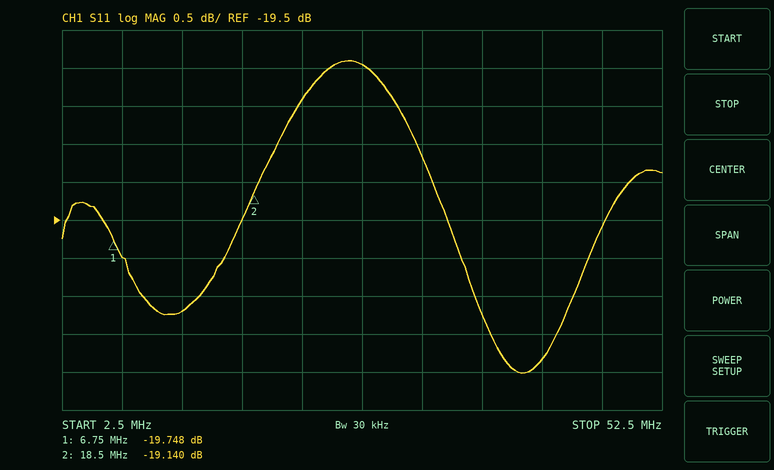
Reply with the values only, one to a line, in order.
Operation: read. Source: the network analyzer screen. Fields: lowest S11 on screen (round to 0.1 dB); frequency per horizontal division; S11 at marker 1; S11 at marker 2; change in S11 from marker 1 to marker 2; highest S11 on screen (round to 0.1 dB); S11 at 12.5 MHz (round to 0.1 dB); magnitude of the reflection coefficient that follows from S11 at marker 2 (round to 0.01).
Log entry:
-21.5 dB
5 MHz
-19.748 dB
-19.140 dB
0.608 dB
-17.4 dB
-20.7 dB
0.11
